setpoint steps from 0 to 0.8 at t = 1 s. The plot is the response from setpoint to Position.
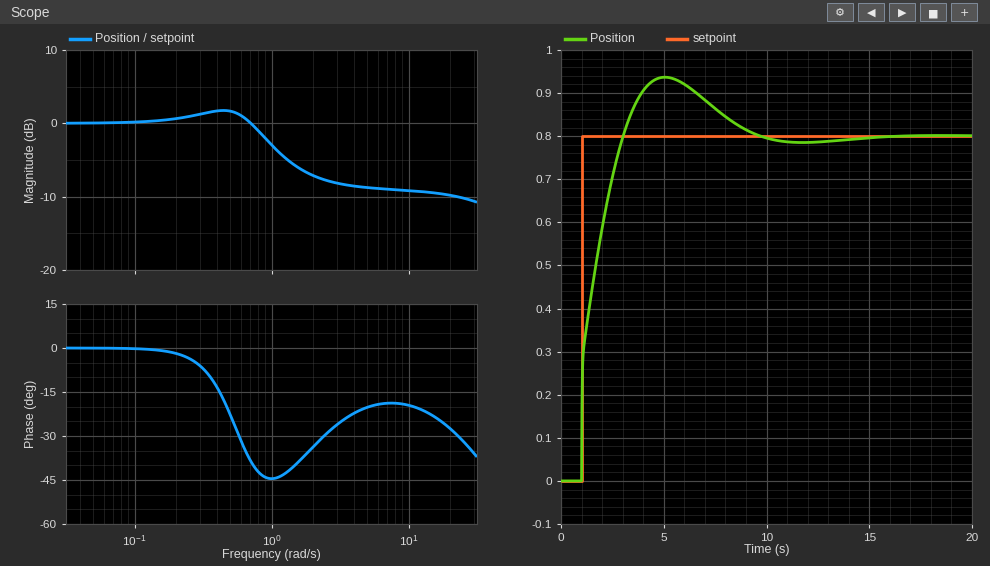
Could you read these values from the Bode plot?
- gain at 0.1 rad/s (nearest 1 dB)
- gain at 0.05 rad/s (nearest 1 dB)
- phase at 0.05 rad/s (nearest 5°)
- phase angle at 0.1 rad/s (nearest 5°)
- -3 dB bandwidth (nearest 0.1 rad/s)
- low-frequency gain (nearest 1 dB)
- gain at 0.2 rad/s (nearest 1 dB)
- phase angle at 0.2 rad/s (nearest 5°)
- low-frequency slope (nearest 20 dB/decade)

0 dB
0 dB
0°
0°
1.0 rad/s
0 dB
1 dB
0°
0 dB/decade
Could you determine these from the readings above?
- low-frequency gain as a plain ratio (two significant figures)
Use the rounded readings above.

1.0
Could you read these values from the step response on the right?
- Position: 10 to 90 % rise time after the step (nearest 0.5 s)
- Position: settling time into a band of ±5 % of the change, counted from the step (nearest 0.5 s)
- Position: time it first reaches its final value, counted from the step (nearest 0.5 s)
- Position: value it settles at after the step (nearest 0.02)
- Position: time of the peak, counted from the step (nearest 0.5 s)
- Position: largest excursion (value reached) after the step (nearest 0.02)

1.5 s
7.0 s
2.0 s
0.80
4.0 s
0.94
